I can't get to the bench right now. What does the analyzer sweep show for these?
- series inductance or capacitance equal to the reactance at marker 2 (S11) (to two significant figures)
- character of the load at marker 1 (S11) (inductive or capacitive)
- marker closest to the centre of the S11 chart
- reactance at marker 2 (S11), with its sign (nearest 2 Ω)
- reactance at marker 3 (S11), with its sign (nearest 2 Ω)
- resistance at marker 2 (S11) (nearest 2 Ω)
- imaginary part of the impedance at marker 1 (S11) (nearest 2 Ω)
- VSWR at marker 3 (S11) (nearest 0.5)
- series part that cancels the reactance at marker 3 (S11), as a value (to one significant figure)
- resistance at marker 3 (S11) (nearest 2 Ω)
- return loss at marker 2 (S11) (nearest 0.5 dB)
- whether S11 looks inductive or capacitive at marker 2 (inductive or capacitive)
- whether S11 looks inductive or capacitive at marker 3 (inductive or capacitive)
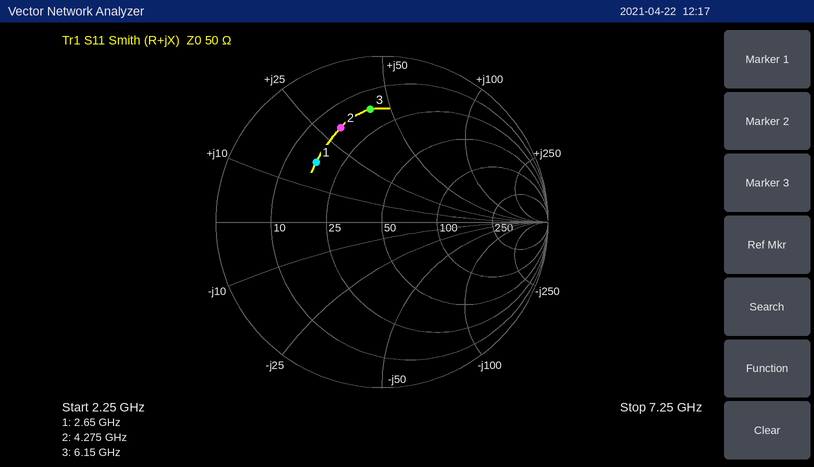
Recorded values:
1.1 nH
inductive
marker 1
+30 Ω
+42 Ω
16 Ω
+18 Ω
5.5
600 fF
16 Ω
4.0 dB
inductive
inductive
